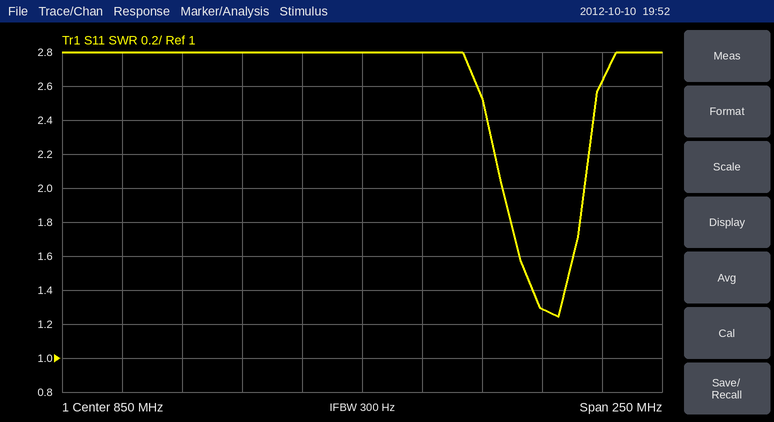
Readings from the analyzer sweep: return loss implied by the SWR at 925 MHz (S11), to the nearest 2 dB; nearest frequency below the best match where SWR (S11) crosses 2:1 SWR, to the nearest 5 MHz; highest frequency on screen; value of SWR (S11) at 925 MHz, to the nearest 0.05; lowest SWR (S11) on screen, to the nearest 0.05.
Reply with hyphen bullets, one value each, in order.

- 18 dB
- 910 MHz
- 975 MHz
- 1.30
- 1.25
